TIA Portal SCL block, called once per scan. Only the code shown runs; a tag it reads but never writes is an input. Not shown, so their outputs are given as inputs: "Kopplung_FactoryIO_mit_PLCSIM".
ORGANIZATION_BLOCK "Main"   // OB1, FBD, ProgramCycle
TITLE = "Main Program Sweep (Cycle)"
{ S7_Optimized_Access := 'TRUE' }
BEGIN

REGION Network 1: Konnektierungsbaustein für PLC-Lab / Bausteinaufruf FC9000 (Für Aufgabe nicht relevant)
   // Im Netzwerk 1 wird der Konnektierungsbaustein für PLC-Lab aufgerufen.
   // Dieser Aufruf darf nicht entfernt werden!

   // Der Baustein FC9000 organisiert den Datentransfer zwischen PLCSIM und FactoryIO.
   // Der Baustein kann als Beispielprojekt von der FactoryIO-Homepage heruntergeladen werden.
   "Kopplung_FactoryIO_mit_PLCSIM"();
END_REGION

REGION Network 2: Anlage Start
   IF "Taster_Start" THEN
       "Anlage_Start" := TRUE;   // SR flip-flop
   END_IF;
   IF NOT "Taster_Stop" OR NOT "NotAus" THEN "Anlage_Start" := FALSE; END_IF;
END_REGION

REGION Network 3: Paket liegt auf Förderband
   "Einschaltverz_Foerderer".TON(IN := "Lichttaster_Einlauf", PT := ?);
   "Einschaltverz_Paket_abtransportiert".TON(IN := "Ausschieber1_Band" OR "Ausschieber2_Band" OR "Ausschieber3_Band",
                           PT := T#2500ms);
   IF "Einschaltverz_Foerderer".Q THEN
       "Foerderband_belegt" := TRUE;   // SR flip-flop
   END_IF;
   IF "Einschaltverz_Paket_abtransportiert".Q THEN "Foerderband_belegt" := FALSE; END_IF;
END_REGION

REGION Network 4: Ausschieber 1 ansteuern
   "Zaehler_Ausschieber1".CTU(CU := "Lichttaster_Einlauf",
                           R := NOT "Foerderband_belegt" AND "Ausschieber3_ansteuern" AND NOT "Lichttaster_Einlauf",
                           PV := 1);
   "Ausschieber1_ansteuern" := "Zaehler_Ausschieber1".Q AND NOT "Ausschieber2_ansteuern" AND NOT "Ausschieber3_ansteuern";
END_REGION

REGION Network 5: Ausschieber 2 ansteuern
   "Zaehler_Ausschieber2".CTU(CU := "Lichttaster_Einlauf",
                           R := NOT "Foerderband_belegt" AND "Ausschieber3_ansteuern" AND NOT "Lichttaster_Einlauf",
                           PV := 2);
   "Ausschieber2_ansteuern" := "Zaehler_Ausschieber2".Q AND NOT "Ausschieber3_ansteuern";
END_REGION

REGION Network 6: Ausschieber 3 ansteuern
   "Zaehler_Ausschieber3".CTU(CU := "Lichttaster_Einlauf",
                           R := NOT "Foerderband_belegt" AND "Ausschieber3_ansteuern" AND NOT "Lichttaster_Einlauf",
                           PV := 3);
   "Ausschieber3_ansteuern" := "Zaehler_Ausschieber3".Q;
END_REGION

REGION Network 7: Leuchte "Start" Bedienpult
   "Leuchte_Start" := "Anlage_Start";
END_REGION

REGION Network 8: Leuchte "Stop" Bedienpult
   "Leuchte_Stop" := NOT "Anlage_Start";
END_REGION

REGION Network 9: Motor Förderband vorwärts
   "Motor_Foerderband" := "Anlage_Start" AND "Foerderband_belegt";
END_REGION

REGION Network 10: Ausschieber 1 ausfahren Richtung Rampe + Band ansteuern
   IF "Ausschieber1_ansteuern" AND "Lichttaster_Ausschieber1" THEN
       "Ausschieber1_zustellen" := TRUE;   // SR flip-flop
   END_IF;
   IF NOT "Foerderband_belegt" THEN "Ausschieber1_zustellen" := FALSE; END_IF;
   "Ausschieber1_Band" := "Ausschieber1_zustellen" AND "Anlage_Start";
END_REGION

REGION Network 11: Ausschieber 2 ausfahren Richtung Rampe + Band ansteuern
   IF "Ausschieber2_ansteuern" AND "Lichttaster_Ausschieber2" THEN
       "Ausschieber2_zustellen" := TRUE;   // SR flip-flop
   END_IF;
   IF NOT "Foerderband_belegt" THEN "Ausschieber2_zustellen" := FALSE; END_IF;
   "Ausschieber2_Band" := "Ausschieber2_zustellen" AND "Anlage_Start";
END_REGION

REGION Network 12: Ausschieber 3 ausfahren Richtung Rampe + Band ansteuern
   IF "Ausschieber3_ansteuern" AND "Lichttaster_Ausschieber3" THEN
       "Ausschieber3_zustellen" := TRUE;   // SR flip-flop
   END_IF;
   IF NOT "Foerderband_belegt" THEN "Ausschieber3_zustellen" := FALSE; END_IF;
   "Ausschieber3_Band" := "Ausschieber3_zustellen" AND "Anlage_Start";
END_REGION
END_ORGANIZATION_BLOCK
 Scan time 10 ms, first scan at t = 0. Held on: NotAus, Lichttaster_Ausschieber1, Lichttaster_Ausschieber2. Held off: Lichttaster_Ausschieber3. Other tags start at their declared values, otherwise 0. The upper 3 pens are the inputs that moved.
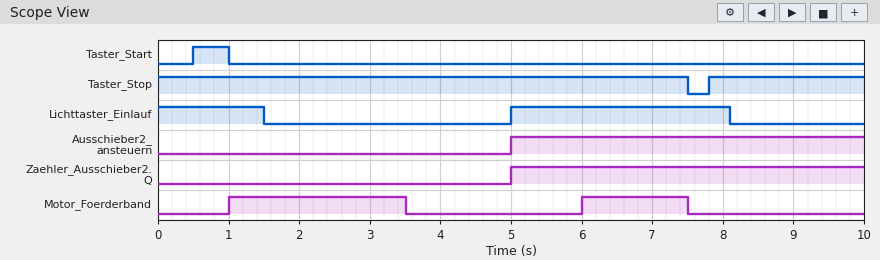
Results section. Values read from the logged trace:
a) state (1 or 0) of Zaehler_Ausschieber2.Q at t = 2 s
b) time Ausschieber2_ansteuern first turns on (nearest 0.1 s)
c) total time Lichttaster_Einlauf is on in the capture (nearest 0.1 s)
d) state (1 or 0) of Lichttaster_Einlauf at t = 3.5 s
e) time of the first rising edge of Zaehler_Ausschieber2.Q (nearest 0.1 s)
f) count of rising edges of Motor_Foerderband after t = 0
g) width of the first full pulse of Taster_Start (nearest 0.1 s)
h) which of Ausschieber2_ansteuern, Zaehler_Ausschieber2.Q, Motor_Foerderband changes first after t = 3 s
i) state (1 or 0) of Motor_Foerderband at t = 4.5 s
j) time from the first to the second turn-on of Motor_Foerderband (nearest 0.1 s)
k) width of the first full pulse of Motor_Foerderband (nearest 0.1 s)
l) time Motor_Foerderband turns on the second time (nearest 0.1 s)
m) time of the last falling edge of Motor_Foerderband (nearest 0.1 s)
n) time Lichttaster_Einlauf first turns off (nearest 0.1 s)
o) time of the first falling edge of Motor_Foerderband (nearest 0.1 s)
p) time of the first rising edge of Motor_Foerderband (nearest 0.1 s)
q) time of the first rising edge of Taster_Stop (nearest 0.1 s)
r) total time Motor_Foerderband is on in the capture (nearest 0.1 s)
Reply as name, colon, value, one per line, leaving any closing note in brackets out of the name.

state (1 or 0) of Zaehler_Ausschieber2.Q at t = 2 s: 0
time Ausschieber2_ansteuern first turns on: 5.0 s
total time Lichttaster_Einlauf is on in the capture: 4.6 s
state (1 or 0) of Lichttaster_Einlauf at t = 3.5 s: 0
time of the first rising edge of Zaehler_Ausschieber2.Q: 5.0 s
count of rising edges of Motor_Foerderband after t = 0: 2
width of the first full pulse of Taster_Start: 0.5 s
which of Ausschieber2_ansteuern, Zaehler_Ausschieber2.Q, Motor_Foerderband changes first after t = 3 s: Motor_Foerderband
state (1 or 0) of Motor_Foerderband at t = 4.5 s: 0
time from the first to the second turn-on of Motor_Foerderband: 5.0 s
width of the first full pulse of Motor_Foerderband: 2.5 s
time Motor_Foerderband turns on the second time: 6.0 s
time of the last falling edge of Motor_Foerderband: 7.5 s
time Lichttaster_Einlauf first turns off: 1.5 s
time of the first falling edge of Motor_Foerderband: 3.5 s
time of the first rising edge of Motor_Foerderband: 1.0 s
time of the first rising edge of Taster_Stop: 7.8 s
total time Motor_Foerderband is on in the capture: 4.0 s
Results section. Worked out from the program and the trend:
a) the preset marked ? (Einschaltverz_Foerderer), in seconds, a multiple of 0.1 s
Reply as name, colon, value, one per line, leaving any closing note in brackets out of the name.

the preset marked ? (Einschaltverz_Foerderer), in seconds, a multiple of 0.1 s: 1.0 s
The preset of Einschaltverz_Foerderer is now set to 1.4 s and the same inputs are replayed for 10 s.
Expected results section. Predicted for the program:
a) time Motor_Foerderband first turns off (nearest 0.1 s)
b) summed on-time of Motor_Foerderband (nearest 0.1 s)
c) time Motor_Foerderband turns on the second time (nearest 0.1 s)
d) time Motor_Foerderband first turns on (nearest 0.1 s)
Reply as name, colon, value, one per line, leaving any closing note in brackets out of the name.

time Motor_Foerderband first turns off: 3.9 s
summed on-time of Motor_Foerderband: 3.6 s
time Motor_Foerderband turns on the second time: 6.4 s
time Motor_Foerderband first turns on: 1.4 s
